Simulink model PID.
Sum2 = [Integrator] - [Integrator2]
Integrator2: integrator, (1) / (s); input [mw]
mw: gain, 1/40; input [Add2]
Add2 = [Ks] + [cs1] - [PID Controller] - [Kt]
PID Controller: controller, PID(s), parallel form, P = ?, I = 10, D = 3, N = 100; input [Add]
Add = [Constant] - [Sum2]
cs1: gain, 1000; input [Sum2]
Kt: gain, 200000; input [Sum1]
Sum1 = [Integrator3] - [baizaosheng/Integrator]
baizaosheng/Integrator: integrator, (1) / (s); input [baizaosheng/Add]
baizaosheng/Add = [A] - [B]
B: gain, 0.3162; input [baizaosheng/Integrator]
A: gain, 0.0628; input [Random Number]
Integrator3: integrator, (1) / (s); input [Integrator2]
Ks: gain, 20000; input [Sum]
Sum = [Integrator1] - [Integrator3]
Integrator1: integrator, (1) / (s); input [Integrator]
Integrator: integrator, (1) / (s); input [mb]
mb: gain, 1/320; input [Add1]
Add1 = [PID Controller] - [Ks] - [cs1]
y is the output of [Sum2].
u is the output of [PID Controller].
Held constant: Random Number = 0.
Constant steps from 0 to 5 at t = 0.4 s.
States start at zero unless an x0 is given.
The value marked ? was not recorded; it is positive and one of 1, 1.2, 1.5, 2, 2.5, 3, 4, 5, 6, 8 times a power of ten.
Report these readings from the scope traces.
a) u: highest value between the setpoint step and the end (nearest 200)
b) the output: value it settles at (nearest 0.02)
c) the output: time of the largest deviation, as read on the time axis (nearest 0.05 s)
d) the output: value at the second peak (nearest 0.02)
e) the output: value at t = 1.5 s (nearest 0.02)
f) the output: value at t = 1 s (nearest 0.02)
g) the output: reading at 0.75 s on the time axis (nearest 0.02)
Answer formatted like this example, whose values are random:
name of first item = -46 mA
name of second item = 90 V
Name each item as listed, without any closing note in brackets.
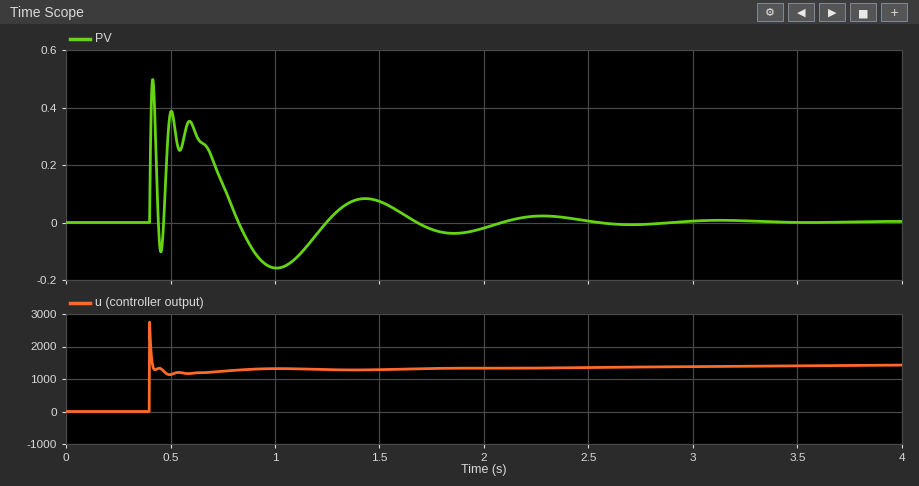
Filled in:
u: highest value between the setpoint step and the end = 2800
the output: value it settles at = 0.00
the output: time of the largest deviation, as read on the time axis = 0.40 s
the output: value at the second peak = 0.38
the output: value at t = 1.5 s = 0.08
the output: value at t = 1 s = -0.16
the output: reading at 0.75 s on the time axis = 0.14
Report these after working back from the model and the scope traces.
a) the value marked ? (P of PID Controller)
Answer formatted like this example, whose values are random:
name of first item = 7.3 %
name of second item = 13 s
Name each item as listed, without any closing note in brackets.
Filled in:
the value marked ? = 250
